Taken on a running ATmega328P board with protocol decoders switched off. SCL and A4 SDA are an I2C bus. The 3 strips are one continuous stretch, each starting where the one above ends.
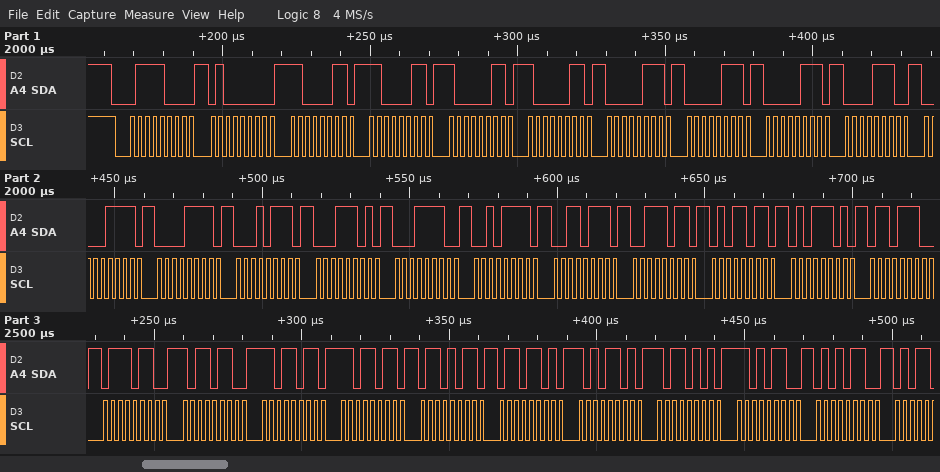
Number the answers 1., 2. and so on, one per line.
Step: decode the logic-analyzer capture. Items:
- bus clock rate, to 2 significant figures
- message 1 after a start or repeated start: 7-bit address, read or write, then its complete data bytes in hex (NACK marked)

1. 400 kHz
2. 0x3C write: 40 C3 C3 83 83 07 07 07 0E 0F 0F 17 1D 1E 2F 37 3B 5B 5D 6E 76 B6 DB DB 6B 6D AD B5 D6 56
